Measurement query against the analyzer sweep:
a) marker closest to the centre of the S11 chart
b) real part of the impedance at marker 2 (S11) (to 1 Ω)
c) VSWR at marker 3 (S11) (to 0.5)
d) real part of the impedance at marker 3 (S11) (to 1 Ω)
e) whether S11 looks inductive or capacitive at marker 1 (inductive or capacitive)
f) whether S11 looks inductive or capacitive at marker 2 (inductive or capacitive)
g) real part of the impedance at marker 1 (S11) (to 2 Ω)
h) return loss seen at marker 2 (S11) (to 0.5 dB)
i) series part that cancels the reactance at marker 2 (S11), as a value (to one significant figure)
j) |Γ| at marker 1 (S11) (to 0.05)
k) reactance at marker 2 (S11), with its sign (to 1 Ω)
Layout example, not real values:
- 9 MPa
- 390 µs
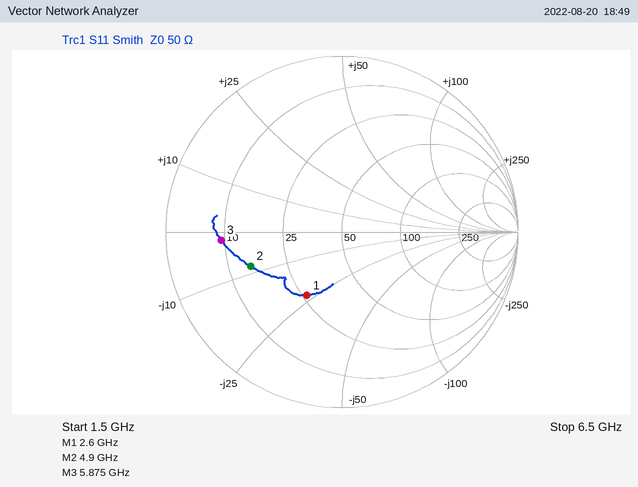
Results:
- marker 1
- 15 Ω
- 5.5
- 9 Ω
- capacitive
- capacitive
- 26 Ω
- 5.0 dB
- 300 pH
- 0.40
- -8 Ω
